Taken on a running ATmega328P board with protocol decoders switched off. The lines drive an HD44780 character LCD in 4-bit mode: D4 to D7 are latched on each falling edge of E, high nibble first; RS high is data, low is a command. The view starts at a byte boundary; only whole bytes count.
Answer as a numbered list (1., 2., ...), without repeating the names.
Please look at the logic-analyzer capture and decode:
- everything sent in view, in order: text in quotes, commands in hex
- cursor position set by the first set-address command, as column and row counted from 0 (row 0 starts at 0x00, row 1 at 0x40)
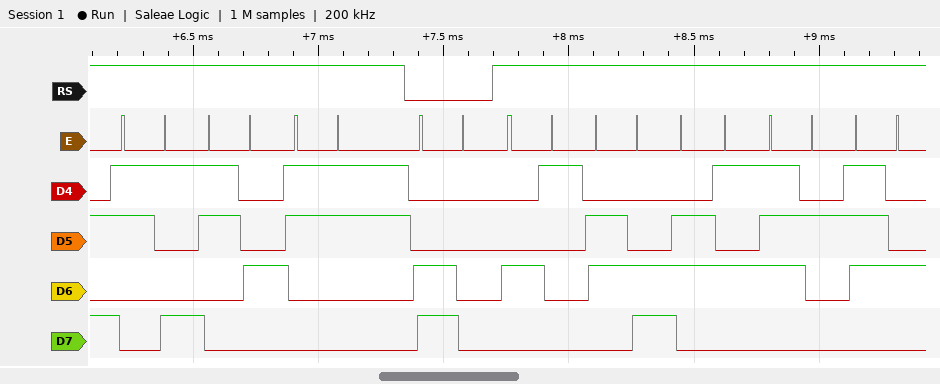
1. "943" 0xC0 "Alert"
2. column 0, row 1
